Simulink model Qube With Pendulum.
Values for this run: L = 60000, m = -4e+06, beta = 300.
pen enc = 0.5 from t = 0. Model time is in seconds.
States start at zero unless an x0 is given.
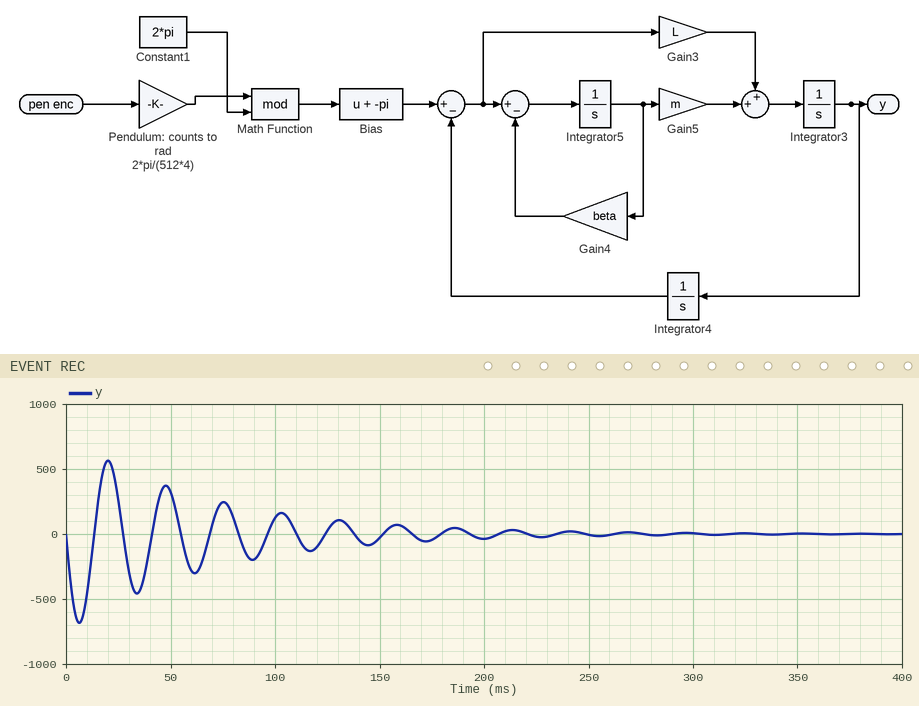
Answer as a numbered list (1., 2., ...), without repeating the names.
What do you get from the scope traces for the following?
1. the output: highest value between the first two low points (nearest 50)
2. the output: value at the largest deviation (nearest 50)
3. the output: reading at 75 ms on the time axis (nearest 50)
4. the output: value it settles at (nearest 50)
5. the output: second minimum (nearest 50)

1. 550
2. -700
3. 250
4. 0
5. -450
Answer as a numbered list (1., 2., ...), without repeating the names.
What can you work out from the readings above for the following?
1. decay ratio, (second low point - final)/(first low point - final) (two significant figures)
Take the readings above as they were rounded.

1. 0.64
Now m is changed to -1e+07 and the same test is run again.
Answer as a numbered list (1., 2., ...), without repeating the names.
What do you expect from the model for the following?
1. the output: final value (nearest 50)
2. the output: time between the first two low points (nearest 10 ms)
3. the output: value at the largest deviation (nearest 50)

1. 0
2. 30 ms
3. -550
